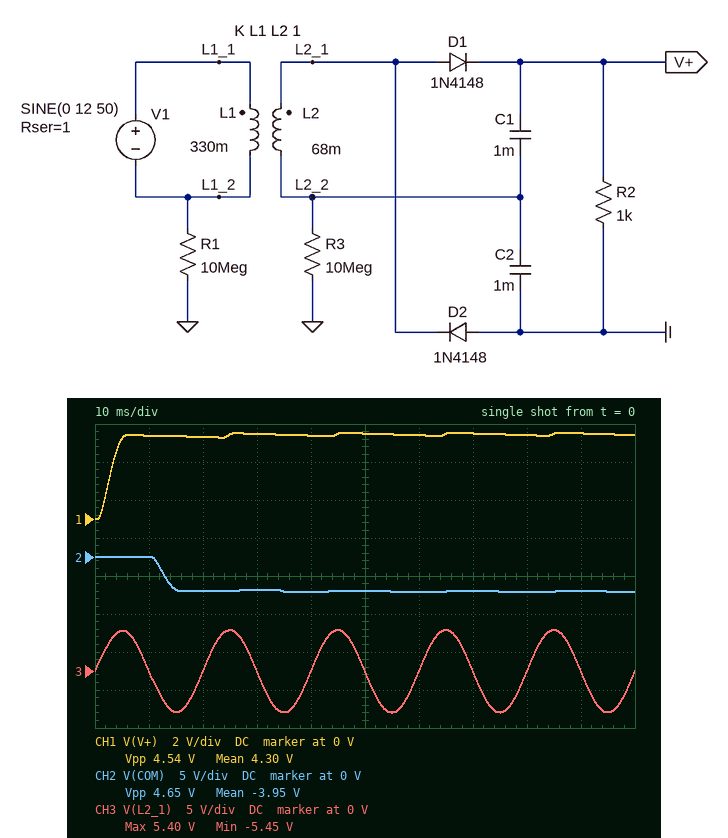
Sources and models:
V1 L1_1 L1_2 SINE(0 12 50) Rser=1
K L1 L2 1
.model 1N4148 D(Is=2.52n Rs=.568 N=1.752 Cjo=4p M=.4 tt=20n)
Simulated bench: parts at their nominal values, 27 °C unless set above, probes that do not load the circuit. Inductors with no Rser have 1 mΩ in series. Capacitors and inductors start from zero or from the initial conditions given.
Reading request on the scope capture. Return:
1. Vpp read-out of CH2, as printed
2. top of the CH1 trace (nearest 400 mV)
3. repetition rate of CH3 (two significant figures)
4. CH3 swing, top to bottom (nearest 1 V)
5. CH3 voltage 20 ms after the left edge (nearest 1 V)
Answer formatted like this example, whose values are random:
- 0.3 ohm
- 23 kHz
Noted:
- 4.65 V
- 4.4 V
- 50 Hz
- 11 V
- 0 V
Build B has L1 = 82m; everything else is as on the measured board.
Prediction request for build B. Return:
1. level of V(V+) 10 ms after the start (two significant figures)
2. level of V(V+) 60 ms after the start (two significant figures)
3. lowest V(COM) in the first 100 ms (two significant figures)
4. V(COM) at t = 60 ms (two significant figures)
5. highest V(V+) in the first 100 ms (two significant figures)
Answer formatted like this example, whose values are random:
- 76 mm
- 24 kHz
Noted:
- 8.8 V
- 9.2 V
- -10 V
- -9.9 V
- 9.6 V
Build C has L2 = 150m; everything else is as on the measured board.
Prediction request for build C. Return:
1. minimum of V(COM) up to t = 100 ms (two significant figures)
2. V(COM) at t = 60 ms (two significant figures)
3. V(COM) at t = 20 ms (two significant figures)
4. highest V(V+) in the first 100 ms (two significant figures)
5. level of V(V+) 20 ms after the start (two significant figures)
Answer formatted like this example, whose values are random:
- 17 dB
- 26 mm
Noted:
- -7.2 V
- -7.1 V
- -6.9 V
- 7.1 V
- 6.6 V
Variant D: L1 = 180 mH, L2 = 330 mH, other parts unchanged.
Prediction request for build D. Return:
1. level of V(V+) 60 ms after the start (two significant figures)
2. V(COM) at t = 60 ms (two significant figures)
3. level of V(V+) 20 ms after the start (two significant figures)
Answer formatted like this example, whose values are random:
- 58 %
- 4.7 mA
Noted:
- 14 V
- -15 V
- 12 V
